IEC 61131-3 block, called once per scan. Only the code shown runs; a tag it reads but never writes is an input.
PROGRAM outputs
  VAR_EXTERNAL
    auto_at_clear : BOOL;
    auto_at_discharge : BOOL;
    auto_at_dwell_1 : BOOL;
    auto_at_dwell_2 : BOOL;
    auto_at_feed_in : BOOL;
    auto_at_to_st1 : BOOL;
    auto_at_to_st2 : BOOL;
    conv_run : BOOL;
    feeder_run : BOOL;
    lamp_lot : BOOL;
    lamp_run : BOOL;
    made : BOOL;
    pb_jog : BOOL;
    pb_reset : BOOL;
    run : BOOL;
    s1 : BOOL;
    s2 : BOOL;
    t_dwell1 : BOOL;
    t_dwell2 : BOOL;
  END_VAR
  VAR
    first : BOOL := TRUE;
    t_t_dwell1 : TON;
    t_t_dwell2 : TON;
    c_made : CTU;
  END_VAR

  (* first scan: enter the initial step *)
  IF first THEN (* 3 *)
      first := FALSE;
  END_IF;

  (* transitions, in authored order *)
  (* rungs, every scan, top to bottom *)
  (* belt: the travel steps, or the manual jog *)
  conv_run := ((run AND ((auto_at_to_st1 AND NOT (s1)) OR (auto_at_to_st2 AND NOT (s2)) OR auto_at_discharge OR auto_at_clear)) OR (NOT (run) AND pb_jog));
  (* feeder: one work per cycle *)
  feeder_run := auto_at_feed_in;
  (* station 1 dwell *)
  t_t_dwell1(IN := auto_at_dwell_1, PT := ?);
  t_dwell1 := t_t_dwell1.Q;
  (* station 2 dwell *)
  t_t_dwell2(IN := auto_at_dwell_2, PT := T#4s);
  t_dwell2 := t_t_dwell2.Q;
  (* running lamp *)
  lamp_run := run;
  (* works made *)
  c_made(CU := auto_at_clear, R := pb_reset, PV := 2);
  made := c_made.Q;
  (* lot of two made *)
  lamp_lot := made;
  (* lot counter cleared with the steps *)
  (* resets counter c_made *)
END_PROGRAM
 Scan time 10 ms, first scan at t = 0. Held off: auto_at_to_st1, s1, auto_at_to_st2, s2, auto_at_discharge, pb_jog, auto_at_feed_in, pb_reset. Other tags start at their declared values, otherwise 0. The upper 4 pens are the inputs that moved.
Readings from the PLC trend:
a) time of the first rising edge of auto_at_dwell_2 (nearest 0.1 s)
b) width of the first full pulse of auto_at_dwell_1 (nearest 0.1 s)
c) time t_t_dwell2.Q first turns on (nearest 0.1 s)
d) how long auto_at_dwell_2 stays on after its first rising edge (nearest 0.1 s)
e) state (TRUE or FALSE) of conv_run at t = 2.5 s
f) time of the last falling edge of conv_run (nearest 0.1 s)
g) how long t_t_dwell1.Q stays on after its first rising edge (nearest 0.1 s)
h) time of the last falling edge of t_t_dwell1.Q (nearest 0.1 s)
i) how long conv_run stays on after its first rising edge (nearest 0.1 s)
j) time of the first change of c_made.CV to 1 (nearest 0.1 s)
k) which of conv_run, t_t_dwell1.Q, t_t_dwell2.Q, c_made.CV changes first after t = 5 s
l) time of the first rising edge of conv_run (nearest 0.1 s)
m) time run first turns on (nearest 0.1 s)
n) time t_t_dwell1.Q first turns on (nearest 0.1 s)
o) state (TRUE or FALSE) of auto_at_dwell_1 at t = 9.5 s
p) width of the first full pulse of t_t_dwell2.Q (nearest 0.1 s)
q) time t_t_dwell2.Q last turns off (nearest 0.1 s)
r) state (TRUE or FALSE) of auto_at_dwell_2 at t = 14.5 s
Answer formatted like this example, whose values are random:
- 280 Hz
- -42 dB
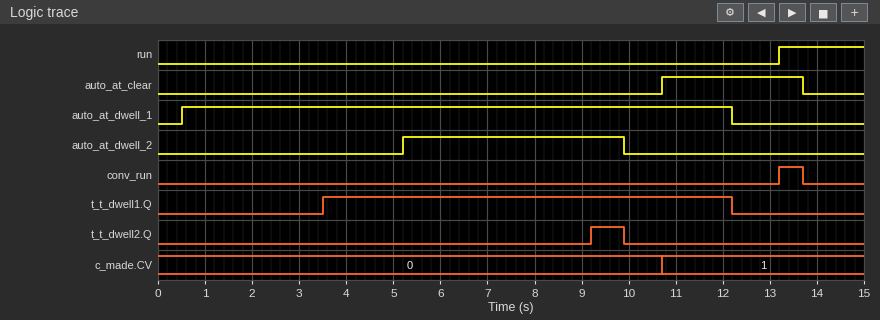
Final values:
- 5.2 s
- 11.7 s
- 9.2 s
- 4.7 s
- FALSE
- 13.7 s
- 8.7 s
- 12.2 s
- 0.5 s
- 10.7 s
- t_t_dwell2.Q
- 13.2 s
- 13.2 s
- 3.5 s
- TRUE
- 0.7 s
- 9.9 s
- FALSE
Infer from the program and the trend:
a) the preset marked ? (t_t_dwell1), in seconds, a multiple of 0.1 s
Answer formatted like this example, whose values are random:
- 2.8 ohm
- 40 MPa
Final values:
- 3.0 s
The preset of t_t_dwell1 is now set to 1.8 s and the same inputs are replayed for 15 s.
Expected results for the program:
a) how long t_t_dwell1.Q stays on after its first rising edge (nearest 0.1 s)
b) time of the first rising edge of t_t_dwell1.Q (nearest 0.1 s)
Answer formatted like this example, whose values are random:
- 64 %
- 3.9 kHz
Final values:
- 9.9 s
- 2.3 s
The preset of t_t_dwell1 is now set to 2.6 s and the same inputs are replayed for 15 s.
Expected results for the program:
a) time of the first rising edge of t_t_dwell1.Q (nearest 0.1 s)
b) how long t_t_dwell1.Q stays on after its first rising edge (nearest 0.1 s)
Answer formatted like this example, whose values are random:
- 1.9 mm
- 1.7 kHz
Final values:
- 3.1 s
- 9.1 s
